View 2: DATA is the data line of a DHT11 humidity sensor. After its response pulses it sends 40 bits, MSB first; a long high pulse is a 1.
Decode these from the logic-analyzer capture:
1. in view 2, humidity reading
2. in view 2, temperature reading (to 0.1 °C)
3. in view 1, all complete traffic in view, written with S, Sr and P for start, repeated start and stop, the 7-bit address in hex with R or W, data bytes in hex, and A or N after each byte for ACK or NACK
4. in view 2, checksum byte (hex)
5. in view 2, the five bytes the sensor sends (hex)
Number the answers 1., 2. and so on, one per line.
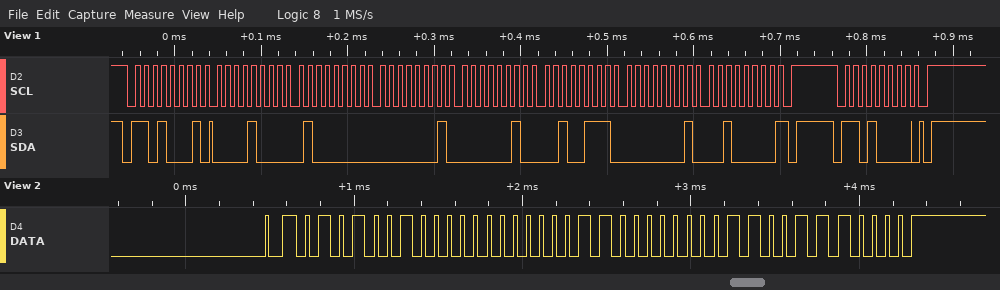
1. 82 %
2. 24.6 °C
3. S 68R A 08 A 40 A 01 A 02 A 27 A 01 A 20 N P S 68W A P
4. 0x70
5. 52 00 18 06 70
